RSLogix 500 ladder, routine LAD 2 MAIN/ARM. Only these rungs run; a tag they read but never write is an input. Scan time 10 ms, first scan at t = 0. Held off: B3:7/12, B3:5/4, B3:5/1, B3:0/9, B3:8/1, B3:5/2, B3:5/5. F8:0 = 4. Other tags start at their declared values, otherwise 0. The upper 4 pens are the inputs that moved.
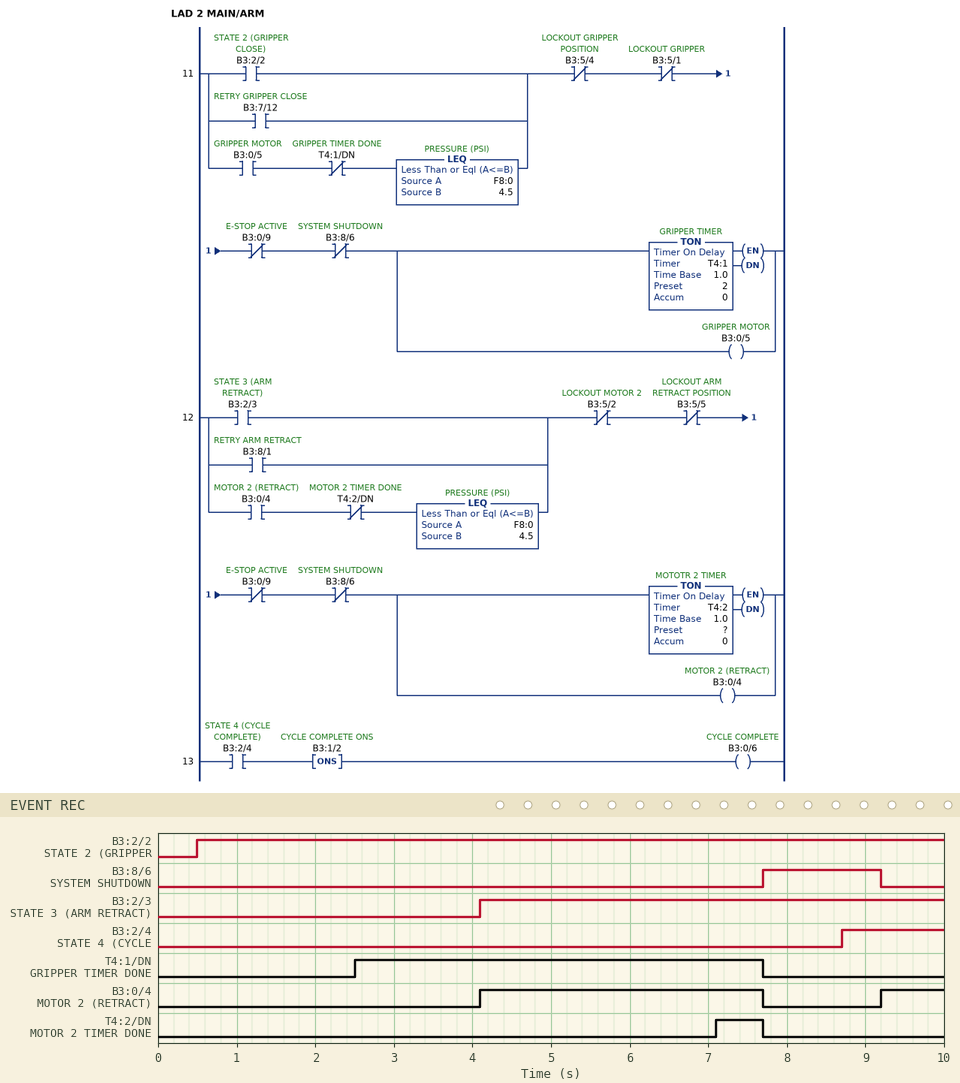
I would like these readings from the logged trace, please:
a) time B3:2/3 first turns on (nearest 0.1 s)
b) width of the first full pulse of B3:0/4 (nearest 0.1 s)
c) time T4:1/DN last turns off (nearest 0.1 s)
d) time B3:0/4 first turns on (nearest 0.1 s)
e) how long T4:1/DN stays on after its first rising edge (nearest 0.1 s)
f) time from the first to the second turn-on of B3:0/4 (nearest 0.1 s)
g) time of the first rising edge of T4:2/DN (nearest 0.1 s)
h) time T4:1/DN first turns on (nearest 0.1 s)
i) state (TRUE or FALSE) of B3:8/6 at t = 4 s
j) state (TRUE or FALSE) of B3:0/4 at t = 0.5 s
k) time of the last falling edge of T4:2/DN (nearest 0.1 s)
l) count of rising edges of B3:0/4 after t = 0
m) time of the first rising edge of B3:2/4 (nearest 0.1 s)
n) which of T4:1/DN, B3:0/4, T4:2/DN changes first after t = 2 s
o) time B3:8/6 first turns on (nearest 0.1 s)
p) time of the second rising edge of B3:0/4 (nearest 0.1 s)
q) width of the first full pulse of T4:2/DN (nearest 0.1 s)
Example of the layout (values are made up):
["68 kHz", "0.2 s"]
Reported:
["4.1 s", "3.6 s", "7.7 s", "4.1 s", "5.2 s", "5.1 s", "7.1 s", "2.5 s", "FALSE", "FALSE", "7.7 s", "2", "8.7 s", "T4:1/DN", "7.7 s", "9.2 s", "0.6 s"]
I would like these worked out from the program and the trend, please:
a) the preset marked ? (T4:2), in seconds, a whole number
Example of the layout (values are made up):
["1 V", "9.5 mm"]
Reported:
["3 s"]
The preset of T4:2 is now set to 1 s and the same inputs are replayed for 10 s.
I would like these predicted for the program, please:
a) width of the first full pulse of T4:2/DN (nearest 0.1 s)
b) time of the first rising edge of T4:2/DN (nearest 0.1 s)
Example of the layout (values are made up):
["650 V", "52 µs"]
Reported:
["2.6 s", "5.1 s"]
